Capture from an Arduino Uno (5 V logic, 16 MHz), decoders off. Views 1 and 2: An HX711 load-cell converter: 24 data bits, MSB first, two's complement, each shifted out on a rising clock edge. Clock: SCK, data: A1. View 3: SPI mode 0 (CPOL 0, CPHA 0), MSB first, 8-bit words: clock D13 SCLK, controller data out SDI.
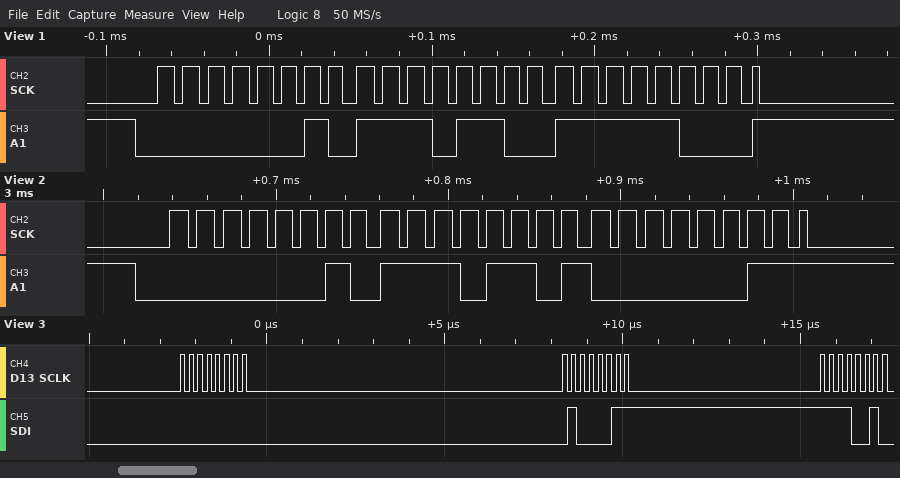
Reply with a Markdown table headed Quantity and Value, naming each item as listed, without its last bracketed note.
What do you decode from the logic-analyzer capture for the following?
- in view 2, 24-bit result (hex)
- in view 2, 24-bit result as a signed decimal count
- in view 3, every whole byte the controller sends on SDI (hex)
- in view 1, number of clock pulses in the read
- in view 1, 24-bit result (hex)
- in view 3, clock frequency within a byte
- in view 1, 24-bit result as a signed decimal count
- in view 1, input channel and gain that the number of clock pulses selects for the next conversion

| Quantity | Value |
|---|---|
| in view 2, 24-bit result | 0x02ED03 |
| in view 2, 24-bit result as a signed decimal count | 191747 |
| in view 3, every whole byte the controller sends on SDI | 00 43 F2 |
| in view 1, number of clock pulses in the read | 25 |
| in view 1, 24-bit result | 0x02ECF8 |
| in view 3, clock frequency within a byte | 4 MHz |
| in view 1, 24-bit result as a signed decimal count | 191736 |
| in view 1, input channel and gain that the number of clock pulses selects for the next conversion | channel A, gain 128 |
